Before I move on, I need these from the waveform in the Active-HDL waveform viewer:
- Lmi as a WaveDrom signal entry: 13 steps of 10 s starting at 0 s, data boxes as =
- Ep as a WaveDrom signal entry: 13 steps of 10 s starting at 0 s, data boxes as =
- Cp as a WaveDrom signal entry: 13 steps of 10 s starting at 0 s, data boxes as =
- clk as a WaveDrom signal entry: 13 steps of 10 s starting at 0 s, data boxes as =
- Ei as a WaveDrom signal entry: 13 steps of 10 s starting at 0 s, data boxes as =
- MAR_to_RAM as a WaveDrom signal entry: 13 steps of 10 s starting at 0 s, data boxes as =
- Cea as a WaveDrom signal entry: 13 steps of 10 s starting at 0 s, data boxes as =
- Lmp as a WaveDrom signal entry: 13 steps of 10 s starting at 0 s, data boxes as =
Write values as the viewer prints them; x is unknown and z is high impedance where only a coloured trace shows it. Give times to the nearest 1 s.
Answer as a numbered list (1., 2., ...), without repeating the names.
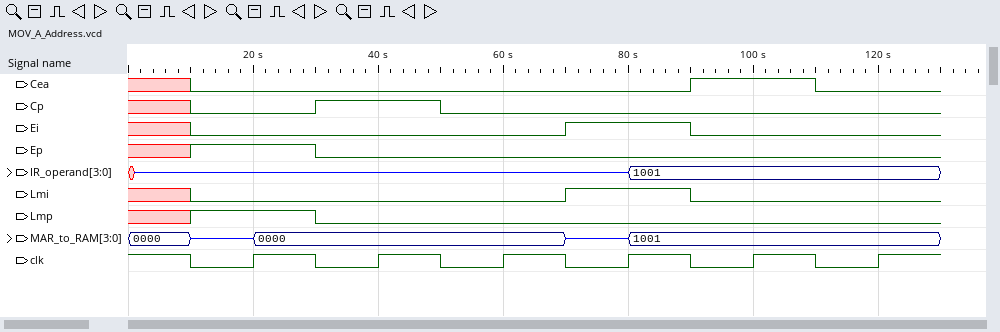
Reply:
1. {name: 'Lmi', wave: 'x0.....1.0...'}
2. {name: 'Ep', wave: 'x1.0.........'}
3. {name: 'Cp', wave: 'x0.1.0.......'}
4. {name: 'clk', wave: '1010101010101'}
5. {name: 'Ei', wave: 'x0.....1.0...'}
6. {name: 'MAR_to_RAM', wave: '=z=....z=....', data: '0000 0000 1001'}
7. {name: 'Cea', wave: 'x0.......1.0.'}
8. {name: 'Lmp', wave: 'x1.0.........'}
